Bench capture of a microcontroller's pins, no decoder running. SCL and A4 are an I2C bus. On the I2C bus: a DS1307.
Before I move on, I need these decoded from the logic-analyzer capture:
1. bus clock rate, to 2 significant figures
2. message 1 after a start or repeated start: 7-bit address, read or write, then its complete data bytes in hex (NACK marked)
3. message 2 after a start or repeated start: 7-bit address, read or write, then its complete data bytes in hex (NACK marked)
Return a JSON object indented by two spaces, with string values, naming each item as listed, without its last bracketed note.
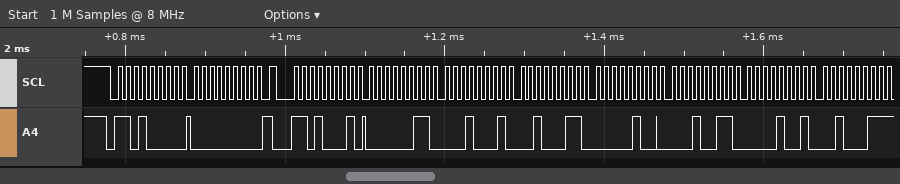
{
  "bus clock rate, to 2 significant figures": "100 kHz",
  "message 1 after a start or repeated start: 7-bit address, read or write, then its complete data bytes in hex": "0x68 write: 00",
  "message 2 after a start or repeated start: 7-bit address, read or write, then its complete data bytes in hex": "0x68 read: 03 11 23 04 13 09 23 NACK"
}
